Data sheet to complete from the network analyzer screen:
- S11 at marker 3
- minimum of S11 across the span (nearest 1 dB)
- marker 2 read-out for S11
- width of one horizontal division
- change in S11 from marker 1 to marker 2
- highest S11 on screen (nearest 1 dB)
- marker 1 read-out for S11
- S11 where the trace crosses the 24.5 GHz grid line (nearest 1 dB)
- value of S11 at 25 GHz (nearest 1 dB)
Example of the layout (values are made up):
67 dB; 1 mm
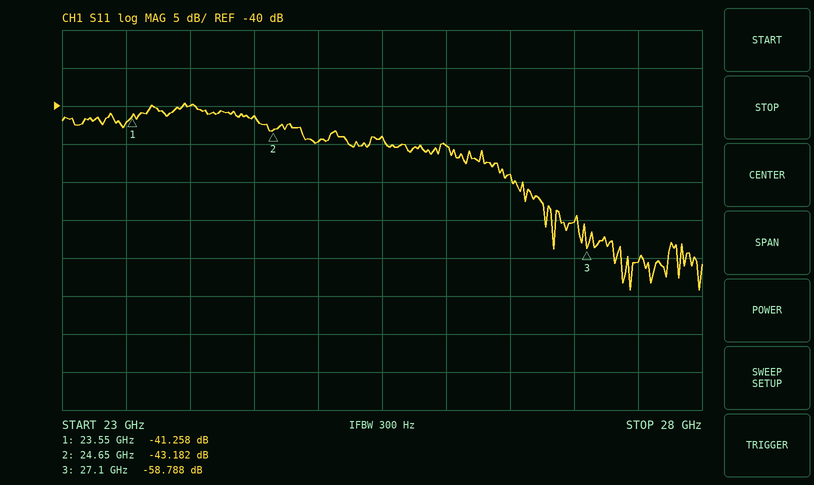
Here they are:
-58.788 dB; -64 dB; -43.182 dB; 500 MHz; -1.924 dB; -40 dB; -41.258 dB; -41 dB; -45 dB
